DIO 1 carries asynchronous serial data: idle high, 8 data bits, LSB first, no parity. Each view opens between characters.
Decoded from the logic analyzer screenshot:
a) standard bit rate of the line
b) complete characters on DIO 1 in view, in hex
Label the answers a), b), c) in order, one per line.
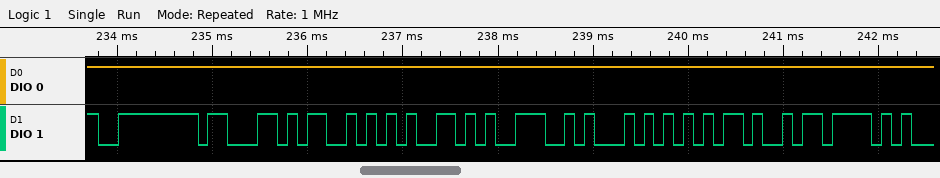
a) 9600 baud
b) FE, 63, 53, 59, 4E, 54, 2D, 7B
